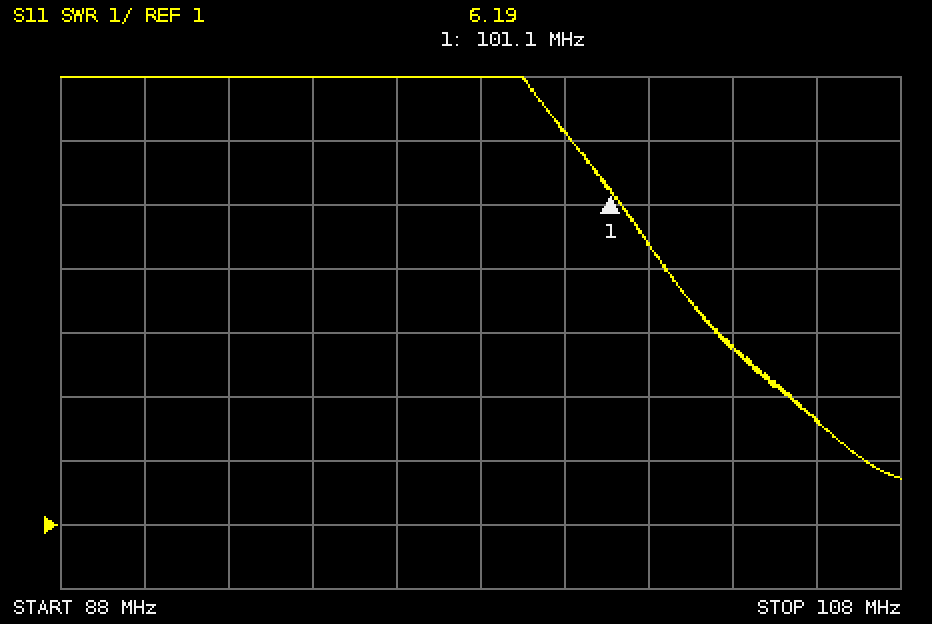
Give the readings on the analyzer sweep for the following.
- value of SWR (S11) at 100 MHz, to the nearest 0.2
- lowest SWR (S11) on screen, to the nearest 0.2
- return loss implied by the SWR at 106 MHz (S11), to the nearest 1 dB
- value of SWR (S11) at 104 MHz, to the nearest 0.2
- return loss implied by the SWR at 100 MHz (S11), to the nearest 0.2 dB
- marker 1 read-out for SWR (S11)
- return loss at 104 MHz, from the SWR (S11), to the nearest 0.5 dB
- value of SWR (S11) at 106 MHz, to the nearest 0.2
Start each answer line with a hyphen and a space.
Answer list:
- 7.2
- 1.8
- 7 dB
- 3.8
- 2.4 dB
- 6.19
- 4.5 dB
- 2.6
